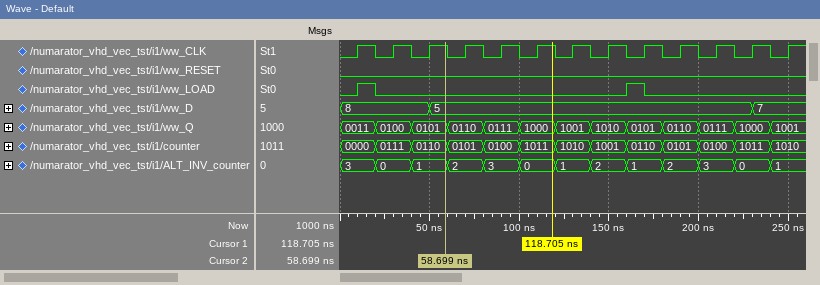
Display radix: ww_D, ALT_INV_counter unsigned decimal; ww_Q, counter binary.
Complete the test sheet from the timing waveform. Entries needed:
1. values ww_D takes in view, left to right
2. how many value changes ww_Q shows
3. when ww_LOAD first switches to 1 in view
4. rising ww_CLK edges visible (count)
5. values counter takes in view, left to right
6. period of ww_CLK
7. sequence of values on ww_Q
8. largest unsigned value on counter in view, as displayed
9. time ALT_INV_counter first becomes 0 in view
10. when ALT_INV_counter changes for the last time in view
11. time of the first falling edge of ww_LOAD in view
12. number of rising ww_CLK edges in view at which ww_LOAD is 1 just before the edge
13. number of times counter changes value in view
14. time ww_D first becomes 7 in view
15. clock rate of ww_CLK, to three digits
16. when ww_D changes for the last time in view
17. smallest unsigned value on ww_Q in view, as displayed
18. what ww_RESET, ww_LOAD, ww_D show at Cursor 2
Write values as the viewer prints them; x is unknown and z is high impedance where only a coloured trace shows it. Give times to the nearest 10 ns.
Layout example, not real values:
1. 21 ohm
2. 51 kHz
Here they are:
1. 8, 5, 7
2. 12
3. 10 ns
4. 13
5. 0000, 0111, 0110, 0101, 0100, 1011, 1010, 1001, 0110, 0101, 0100, 1011, 1010
6. 20 ns
7. 0011, 0100, 0101, 0110, 0111, 1000, 1001, 1010, 0101, 0110, 0111, 1000, 1001
8. 1011
9. 20 ns
10. 240 ns
11. 20 ns
12. 1
13. 12
14. 230 ns
15. 50.0 MHz
16. 230 ns
17. 0011
18. ww_RESET=0, ww_LOAD=0, ww_D=5
